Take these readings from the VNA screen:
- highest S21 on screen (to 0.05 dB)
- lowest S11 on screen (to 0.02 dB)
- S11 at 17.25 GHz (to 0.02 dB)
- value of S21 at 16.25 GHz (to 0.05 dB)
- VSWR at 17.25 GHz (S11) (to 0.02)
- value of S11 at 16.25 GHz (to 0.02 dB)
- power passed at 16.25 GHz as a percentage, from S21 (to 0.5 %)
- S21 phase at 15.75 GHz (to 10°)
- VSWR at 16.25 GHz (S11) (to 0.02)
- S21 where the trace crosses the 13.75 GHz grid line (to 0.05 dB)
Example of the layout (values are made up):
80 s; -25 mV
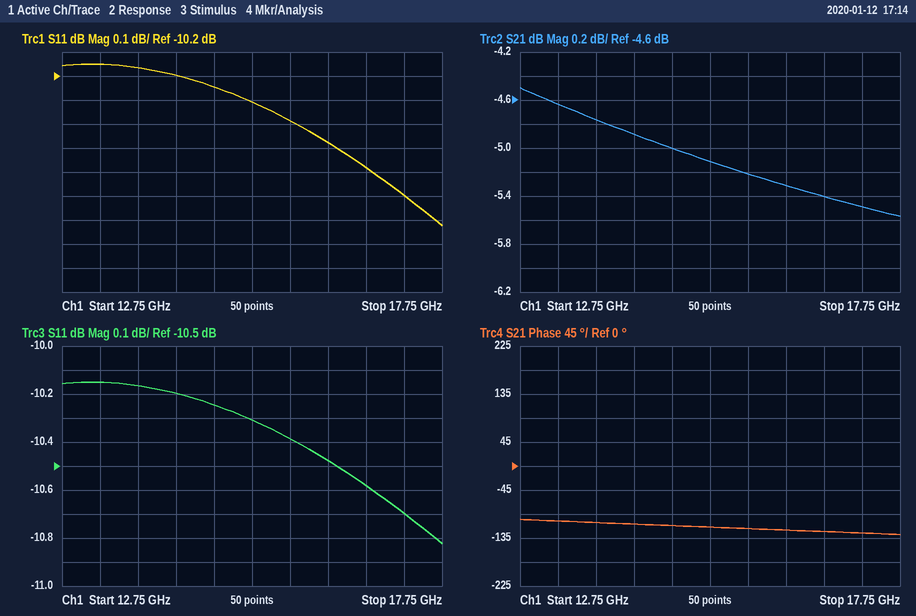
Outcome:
-4.50 dB; -10.82 dB; -10.70 dB; -5.30 dB; 1.82; -10.48 dB; 29.5 %; -120°; 1.86; -4.75 dB
